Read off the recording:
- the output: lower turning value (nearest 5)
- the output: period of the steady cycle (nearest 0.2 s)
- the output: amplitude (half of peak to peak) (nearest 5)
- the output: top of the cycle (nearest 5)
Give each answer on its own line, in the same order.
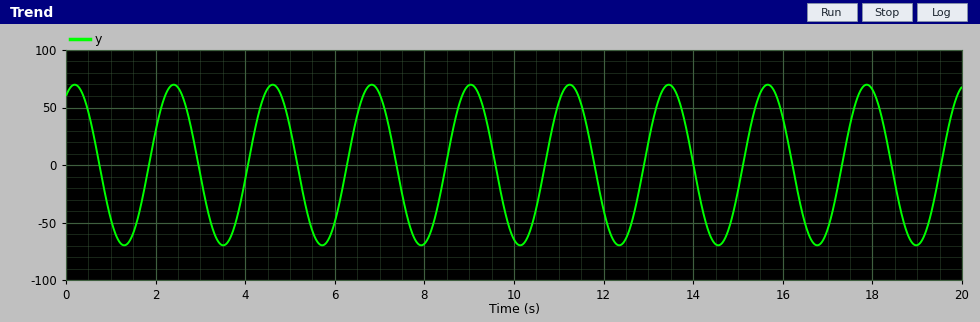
-70
2.2 s
70
70
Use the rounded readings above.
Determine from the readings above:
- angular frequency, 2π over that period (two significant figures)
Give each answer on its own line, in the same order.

2.9 rad/s
